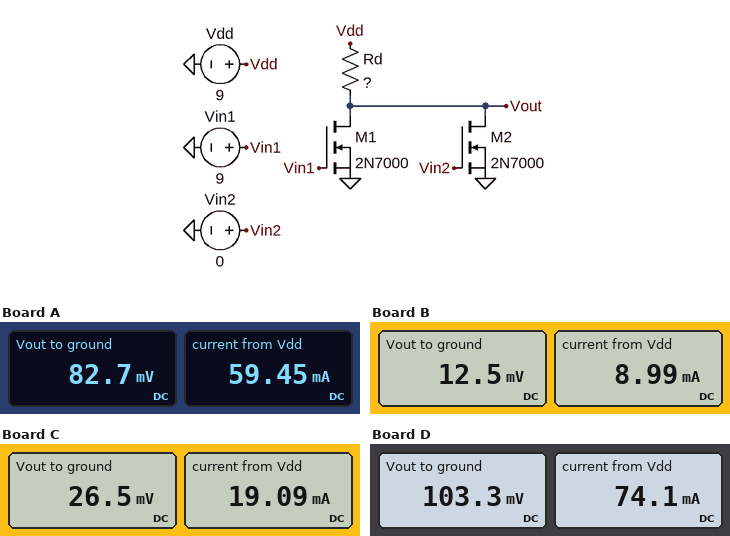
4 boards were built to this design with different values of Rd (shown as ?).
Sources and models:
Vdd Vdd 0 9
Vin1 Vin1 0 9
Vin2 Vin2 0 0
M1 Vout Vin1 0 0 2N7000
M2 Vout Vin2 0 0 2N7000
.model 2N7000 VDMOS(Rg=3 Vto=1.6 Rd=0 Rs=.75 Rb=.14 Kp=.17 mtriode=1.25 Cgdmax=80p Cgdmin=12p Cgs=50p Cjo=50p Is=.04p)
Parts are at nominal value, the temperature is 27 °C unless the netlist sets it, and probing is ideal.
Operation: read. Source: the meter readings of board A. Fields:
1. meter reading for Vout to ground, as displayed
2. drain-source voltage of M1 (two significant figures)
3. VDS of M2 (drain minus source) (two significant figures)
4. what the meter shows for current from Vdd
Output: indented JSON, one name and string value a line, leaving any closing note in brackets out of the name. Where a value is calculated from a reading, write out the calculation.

{
  "meter reading for Vout to ground, as displayed": "82.7 mV",
  "drain-source voltage of M1": "82.7 mV = 83 mV",
  "VDS of M2 (drain minus source)": "82.7 mV = 83 mV",
  "what the meter shows for current from Vdd": "59.45 mA"
}
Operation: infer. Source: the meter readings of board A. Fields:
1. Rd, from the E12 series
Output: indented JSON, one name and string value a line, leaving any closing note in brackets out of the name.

{
  "Rd, from the E12 series": "150 Ω"
}
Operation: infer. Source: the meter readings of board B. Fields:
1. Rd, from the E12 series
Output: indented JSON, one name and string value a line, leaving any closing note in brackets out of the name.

{
  "Rd, from the E12 series": "1 kΩ"
}
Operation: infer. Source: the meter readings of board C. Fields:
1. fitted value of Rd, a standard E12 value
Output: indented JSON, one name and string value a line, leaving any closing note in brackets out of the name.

{
  "fitted value of Rd, a standard E12 value": "470 Ω"
}
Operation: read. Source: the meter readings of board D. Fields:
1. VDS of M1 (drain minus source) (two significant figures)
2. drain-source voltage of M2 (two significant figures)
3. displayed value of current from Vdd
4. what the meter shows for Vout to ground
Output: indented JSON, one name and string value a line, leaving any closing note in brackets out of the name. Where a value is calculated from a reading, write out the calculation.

{
  "VDS of M1 (drain minus source)": "103.3 mV = 100 mV",
  "drain-source voltage of M2": "103.3 mV = 100 mV",
  "displayed value of current from Vdd": "74.1 mA",
  "what the meter shows for Vout to ground": "103.3 mV"
}
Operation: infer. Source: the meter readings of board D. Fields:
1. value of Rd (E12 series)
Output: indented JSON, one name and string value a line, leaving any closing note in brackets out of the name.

{
  "value of Rd": "120 Ω"
}
